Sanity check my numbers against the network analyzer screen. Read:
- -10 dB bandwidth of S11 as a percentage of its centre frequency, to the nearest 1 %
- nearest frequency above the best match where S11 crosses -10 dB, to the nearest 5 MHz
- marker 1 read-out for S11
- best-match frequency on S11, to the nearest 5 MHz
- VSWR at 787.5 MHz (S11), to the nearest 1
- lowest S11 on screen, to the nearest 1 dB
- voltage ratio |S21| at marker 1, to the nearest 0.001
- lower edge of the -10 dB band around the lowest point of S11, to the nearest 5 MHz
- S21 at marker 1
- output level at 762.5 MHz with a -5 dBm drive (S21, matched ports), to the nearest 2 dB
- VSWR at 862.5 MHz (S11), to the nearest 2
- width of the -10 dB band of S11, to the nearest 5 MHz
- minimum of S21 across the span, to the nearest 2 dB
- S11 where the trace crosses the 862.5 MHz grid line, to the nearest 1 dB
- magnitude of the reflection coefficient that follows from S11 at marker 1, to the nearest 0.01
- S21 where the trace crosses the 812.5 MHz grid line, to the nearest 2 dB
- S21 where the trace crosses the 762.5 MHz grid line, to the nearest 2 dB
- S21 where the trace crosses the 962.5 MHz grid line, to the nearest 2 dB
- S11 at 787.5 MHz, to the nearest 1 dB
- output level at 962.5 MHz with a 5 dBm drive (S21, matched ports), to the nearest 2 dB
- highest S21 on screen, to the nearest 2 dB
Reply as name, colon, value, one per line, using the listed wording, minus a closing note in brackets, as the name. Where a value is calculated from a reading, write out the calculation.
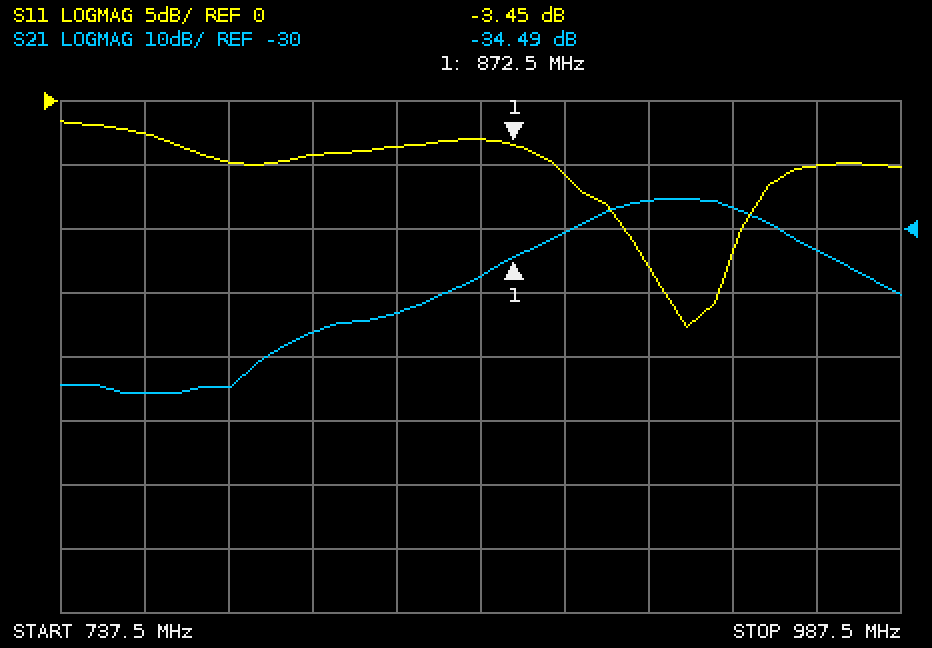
-10 dB bandwidth of S11 as a percentage of its centre frequency, to the nearest 1 %: 35 MHz / 922.5 MHz ≈ 4 %
nearest frequency above the best match where S11 crosses -10 dB, to the nearest 5 MHz: 940 MHz
marker 1 read-out for S11: -3.45 dB
best-match frequency on S11, to the nearest 5 MHz: 925 MHz
VSWR at 787.5 MHz (S11), to the nearest 1: |Γ| = 10^(-5/20) = 0.5623; VSWR = (1 + 0.5623)/(1 − 0.5623) ≈ 4
lowest S11 on screen, to the nearest 1 dB: -18 dB
voltage ratio |S21| at marker 1, to the nearest 0.001: 10^(-34.49/20) ≈ 0.019
lower edge of the -10 dB band around the lowest point of S11, to the nearest 5 MHz: 905 MHz
S21 at marker 1: -34.49 dB
output level at 762.5 MHz with a -5 dBm drive (S21, matched ports), to the nearest 2 dB: -5 dBm + (-56 dB) = -60 dBm
VSWR at 862.5 MHz (S11), to the nearest 2: |Γ| = 10^(-3/20) = 0.7079; VSWR = (1 + 0.7079)/(1 − 0.7079) ≈ 6
width of the -10 dB band of S11, to the nearest 5 MHz: 940 MHz − 905 MHz = 35 MHz
minimum of S21 across the span, to the nearest 2 dB: -56 dB
S11 where the trace crosses the 862.5 MHz grid line, to the nearest 1 dB: -3 dB
magnitude of the reflection coefficient that follows from S11 at marker 1, to the nearest 0.01: 10^(-3.45/20) ≈ 0.67
S21 where the trace crosses the 812.5 MHz grid line, to the nearest 2 dB: -46 dB
S21 where the trace crosses the 762.5 MHz grid line, to the nearest 2 dB: -56 dB
S21 where the trace crosses the 962.5 MHz grid line, to the nearest 2 dB: -34 dB
S11 at 787.5 MHz, to the nearest 1 dB: -5 dB
output level at 962.5 MHz with a 5 dBm drive (S21, matched ports), to the nearest 2 dB: 5 dBm + (-34 dB) = -28 dBm
highest S21 on screen, to the nearest 2 dB: -26 dB
